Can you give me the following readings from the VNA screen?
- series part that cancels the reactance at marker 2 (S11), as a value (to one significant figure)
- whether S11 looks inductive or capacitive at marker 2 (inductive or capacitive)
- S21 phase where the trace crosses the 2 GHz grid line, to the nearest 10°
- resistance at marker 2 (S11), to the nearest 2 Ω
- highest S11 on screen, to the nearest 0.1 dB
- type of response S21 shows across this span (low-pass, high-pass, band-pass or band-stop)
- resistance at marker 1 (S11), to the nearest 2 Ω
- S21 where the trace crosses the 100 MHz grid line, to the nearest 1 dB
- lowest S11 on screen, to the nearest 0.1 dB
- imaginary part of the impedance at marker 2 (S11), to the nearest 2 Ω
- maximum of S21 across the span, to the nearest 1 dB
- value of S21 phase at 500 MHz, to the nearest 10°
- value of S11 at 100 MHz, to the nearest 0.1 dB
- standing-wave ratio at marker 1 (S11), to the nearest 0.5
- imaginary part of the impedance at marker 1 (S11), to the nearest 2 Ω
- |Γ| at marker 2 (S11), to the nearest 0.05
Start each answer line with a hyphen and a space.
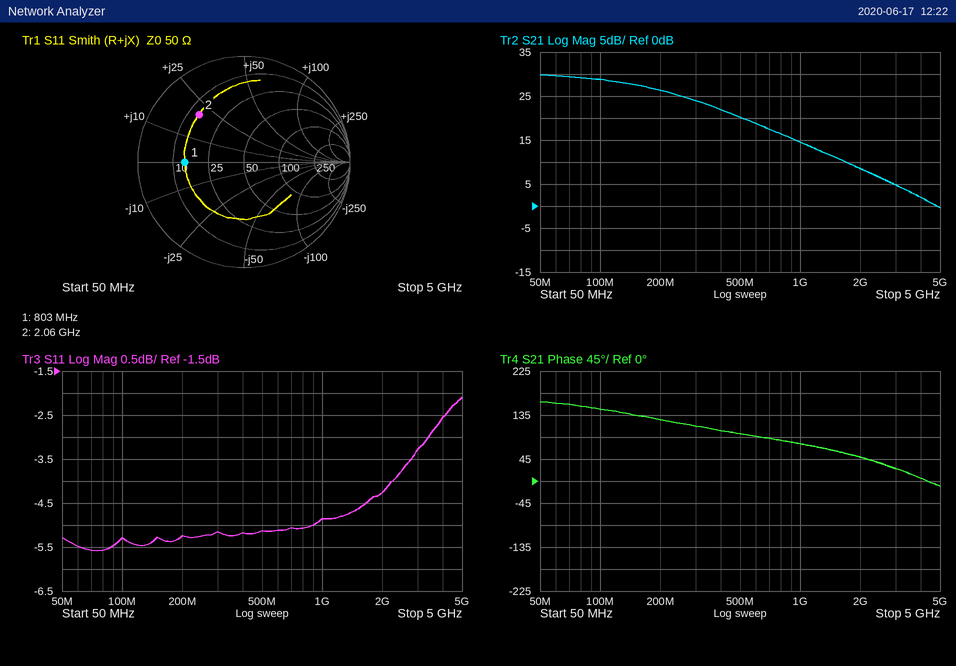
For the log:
- 4 pF
- inductive
- 50°
- 14 Ω
- -2.1 dB
- low-pass
- 14 Ω
- 29 dB
- -5.6 dB
- +20 Ω
- 30 dB
- 100°
- -5.3 dB
- 3.5
- 0 Ω
- 0.60
